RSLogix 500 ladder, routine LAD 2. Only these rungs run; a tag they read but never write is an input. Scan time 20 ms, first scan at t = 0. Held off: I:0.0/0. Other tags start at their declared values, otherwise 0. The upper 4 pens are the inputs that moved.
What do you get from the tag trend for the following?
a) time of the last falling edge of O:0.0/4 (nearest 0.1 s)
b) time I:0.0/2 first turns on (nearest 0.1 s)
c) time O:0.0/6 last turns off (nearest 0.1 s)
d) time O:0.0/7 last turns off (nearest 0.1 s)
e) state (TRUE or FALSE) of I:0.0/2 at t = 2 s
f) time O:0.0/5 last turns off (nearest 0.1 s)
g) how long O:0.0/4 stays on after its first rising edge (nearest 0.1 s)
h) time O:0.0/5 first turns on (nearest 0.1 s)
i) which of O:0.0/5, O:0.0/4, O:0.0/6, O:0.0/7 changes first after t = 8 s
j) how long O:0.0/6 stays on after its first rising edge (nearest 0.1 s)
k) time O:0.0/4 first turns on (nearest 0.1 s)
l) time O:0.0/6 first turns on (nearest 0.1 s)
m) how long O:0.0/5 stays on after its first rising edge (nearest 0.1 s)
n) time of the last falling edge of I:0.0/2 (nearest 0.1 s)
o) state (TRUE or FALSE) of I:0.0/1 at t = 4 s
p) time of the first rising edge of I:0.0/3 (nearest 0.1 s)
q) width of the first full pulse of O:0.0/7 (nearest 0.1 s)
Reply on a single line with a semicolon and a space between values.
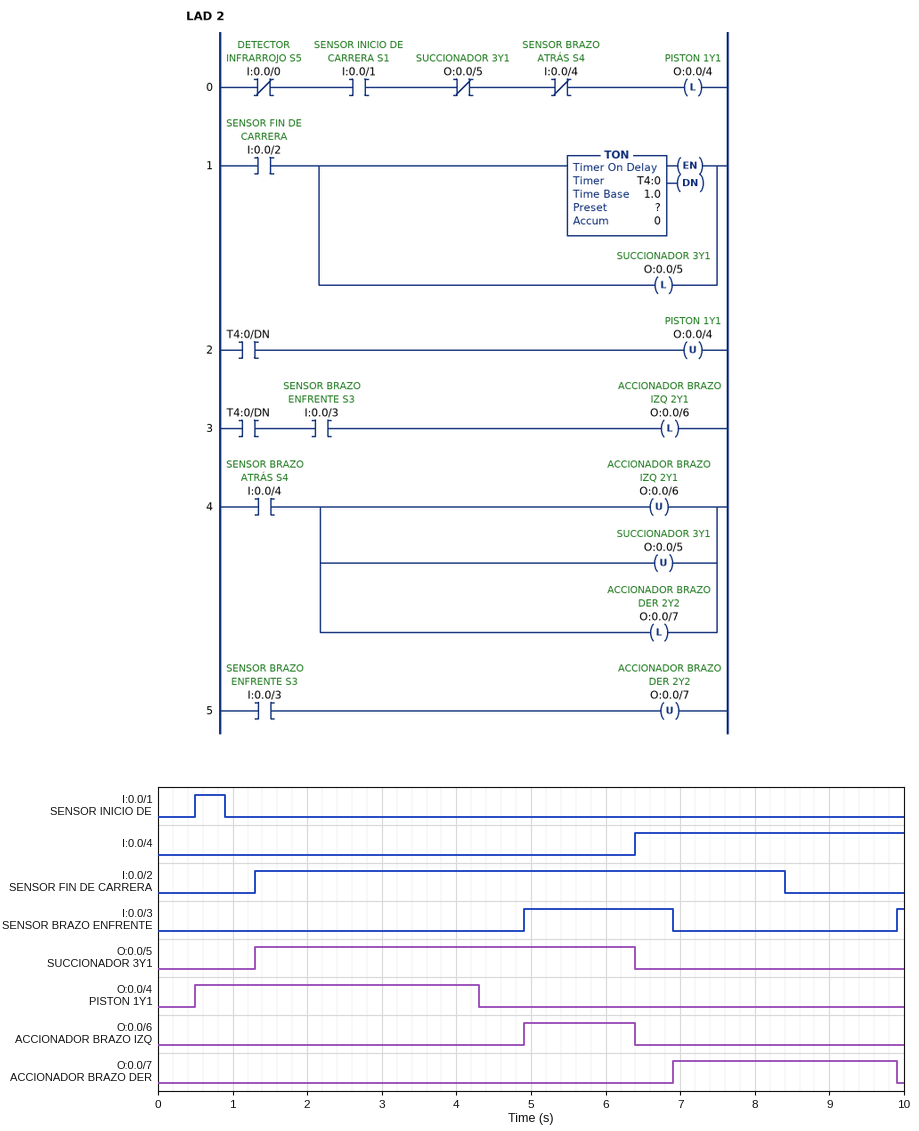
4.3 s; 1.3 s; 6.4 s; 9.9 s; TRUE; 6.4 s; 3.8 s; 1.3 s; O:0.0/7; 1.5 s; 0.5 s; 4.9 s; 5.1 s; 8.4 s; FALSE; 4.9 s; 3.0 s
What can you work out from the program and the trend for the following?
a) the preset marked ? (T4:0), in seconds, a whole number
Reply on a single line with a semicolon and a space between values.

3 s
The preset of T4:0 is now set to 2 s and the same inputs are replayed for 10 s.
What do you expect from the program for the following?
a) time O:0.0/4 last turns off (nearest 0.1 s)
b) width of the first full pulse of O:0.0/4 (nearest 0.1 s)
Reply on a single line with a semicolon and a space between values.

3.3 s; 2.8 s
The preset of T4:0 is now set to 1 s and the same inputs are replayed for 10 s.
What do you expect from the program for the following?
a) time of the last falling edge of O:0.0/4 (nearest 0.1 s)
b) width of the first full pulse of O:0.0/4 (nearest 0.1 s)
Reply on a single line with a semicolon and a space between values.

2.3 s; 1.8 s
